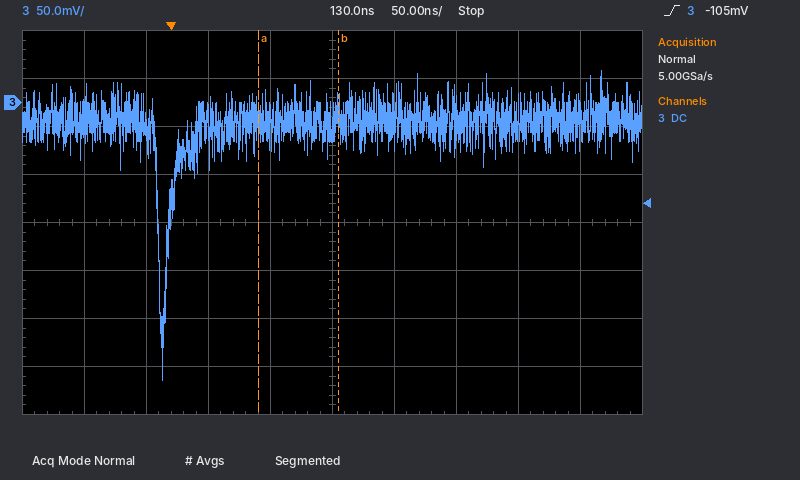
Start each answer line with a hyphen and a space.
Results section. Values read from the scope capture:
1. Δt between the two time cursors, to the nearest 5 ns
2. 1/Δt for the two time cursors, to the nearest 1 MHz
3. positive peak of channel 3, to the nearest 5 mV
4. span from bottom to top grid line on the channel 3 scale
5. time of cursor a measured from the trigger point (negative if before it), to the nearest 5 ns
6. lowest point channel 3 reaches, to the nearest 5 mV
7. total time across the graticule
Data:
- 65 ns
- 15 MHz
- 35 mV
- 400 mV
- +70 ns
- -290 mV
- 500 ns
